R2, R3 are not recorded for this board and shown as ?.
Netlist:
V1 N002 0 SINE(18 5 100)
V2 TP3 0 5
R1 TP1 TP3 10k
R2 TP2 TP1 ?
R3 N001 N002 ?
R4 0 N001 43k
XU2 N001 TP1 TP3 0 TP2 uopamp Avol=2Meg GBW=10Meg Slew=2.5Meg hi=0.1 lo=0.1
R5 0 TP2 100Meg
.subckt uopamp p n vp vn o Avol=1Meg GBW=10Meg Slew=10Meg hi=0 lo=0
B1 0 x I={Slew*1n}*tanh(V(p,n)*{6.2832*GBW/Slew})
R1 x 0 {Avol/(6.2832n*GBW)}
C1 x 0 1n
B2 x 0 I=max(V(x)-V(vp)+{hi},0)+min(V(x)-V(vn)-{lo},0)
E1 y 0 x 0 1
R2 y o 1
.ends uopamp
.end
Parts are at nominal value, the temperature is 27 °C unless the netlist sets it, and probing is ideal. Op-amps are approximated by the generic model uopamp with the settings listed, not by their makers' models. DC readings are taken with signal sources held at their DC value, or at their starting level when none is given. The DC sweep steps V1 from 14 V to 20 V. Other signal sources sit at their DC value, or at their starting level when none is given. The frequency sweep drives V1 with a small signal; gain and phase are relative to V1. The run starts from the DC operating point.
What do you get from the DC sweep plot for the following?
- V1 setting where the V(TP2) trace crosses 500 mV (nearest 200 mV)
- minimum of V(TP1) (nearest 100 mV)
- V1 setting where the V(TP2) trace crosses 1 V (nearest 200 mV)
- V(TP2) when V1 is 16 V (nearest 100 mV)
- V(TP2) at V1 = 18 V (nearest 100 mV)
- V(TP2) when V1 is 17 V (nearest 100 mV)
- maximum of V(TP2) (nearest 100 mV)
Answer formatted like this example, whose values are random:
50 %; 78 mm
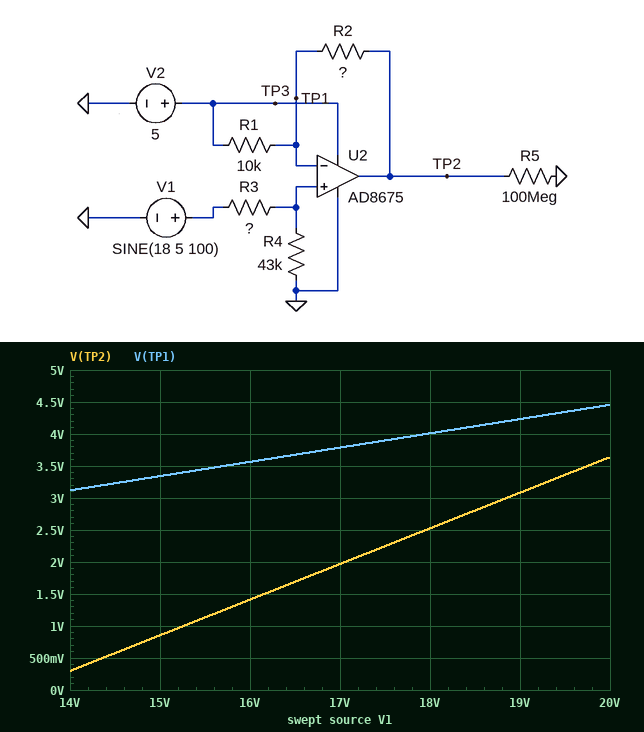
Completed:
14.4 V; 3.1 V; 15.2 V; 1.4 V; 2.5 V; 2.0 V; 3.6 V
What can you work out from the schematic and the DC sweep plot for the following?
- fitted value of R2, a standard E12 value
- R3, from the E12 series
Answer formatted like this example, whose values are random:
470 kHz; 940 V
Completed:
15 kΩ; 150 kΩ
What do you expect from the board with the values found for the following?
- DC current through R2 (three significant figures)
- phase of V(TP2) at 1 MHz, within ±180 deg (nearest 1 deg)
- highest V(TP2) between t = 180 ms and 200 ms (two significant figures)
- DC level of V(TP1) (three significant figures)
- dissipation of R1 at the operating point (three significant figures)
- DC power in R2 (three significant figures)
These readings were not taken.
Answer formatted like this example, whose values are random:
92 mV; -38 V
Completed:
99.0 µA; -14 deg; 4.9 V; 4.01 V; 97.9 µW; 147 µW
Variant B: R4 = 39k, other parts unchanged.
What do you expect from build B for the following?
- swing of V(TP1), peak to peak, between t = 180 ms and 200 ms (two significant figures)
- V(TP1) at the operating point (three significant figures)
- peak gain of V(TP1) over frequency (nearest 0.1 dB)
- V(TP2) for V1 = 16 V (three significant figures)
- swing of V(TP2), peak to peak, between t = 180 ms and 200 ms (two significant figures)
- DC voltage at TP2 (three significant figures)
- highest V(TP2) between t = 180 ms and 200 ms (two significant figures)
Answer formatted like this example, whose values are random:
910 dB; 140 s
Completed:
1.7 V; 3.71 V; -13.7 dB; 754 mV; 4.3 V; 1.79 V; 4.4 V
